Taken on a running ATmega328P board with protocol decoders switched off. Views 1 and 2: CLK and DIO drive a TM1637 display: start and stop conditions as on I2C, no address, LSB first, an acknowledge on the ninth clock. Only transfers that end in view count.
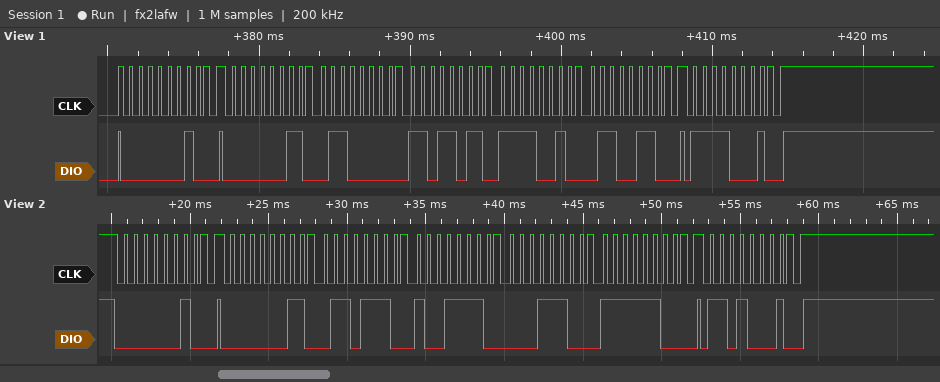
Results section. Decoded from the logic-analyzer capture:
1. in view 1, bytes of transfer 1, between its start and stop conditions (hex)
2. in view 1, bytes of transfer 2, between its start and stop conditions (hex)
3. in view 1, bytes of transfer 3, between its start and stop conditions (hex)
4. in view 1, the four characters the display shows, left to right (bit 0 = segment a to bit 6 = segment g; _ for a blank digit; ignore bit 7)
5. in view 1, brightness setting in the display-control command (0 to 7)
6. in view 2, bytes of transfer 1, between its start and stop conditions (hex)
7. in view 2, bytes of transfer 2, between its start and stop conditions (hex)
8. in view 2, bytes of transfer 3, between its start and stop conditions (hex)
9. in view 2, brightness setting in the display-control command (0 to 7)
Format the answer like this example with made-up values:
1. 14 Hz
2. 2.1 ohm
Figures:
1. 40
2. C0 06 DB 4F 66
3. 8F
4. 1234
5. 7
6. 40
7. C0 76 79 38 3F
8. 8B
9. 3
